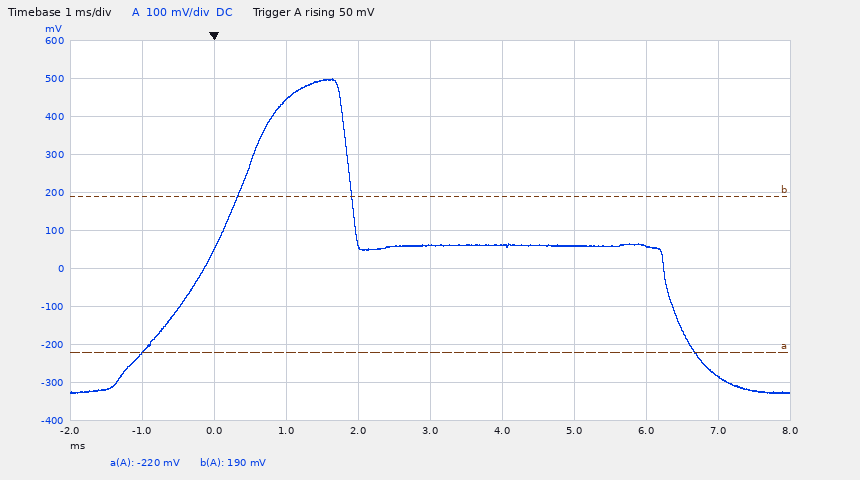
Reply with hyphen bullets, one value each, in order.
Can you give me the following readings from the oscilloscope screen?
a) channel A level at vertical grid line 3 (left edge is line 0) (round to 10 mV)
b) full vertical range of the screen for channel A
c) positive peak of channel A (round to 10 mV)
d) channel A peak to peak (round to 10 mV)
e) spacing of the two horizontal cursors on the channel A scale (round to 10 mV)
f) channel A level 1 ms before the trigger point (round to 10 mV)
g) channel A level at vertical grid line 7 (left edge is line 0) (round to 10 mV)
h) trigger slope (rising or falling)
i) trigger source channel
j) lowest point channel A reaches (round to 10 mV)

- 440 mV
- 1 V
- 500 mV
- 830 mV
- 410 mV
- -220 mV
- 60 mV
- rising
- channel A
- -330 mV
